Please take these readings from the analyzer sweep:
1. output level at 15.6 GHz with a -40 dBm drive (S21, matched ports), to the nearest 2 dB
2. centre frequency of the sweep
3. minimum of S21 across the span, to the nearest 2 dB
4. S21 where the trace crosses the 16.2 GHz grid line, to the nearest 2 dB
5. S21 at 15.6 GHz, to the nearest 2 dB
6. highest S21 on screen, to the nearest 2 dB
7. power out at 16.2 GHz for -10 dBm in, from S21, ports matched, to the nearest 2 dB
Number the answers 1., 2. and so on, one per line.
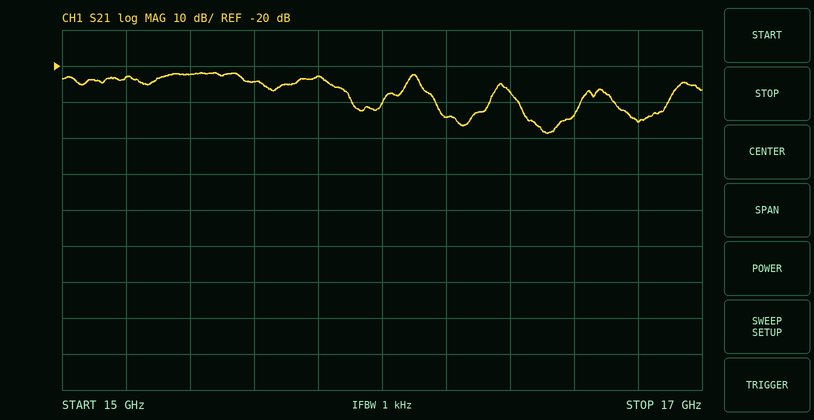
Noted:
1. -64 dBm
2. 16 GHz
3. -38 dB
4. -34 dB
5. -24 dB
6. -22 dB
7. -44 dBm
